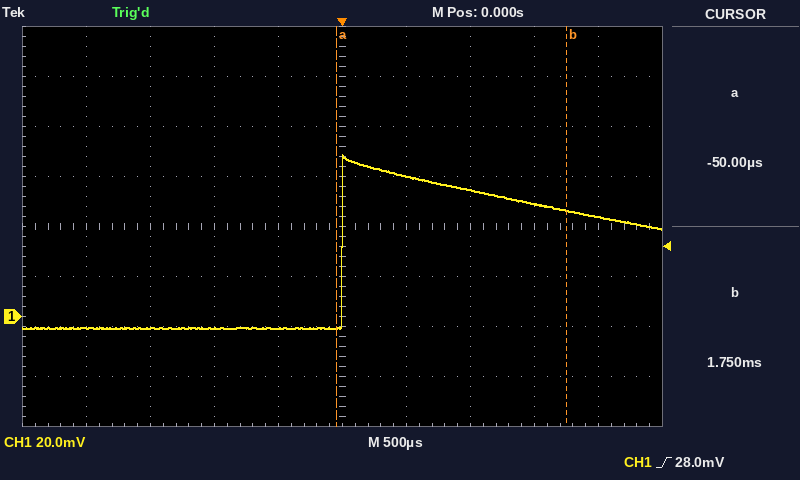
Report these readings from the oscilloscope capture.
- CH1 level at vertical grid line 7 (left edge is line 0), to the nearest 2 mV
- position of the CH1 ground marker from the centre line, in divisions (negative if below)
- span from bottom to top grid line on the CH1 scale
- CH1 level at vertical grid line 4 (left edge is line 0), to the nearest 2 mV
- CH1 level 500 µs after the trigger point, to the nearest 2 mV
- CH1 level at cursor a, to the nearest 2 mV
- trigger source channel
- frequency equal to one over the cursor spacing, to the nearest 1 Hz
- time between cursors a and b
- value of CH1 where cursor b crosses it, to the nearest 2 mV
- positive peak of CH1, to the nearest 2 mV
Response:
50 mV
-1.8 div
160 mV
-4 mV
56 mV
-4 mV
CH1
556 Hz
1.80 ms
42 mV
64 mV
